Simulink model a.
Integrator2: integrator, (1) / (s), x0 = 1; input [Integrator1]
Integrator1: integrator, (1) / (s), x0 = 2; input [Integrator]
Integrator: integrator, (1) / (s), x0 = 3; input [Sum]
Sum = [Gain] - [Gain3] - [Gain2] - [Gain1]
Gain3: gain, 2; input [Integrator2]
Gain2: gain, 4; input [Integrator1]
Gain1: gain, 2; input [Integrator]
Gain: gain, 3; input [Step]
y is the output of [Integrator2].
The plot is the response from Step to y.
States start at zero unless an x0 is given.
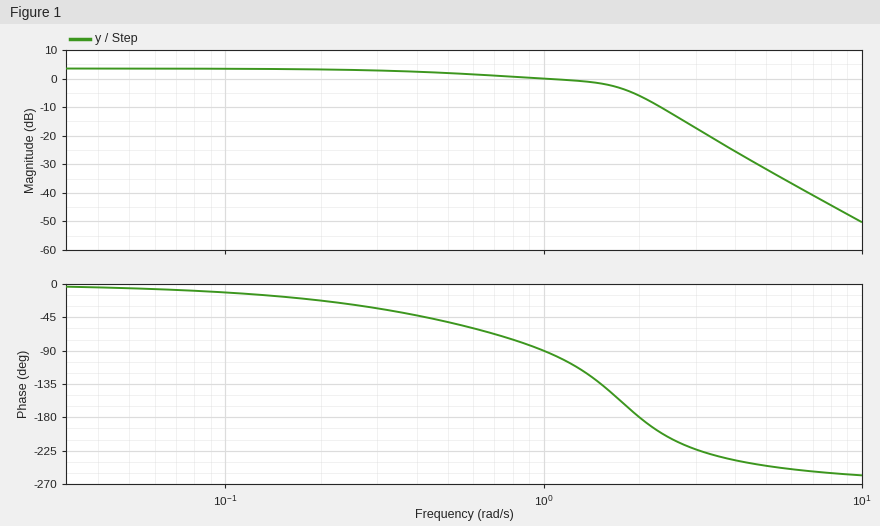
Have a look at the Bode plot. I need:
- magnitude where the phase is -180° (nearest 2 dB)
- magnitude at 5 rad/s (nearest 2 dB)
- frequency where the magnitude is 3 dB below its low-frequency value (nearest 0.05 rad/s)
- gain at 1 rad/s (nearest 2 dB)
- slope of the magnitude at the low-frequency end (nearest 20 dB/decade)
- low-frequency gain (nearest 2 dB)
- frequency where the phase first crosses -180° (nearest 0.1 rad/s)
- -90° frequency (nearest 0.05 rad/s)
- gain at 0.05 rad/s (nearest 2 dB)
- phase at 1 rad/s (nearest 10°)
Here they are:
-6 dB
-32 dB
0.85 rad/s
0 dB
0 dB/decade
4 dB
2.0 rad/s
1.00 rad/s
4 dB
-90°
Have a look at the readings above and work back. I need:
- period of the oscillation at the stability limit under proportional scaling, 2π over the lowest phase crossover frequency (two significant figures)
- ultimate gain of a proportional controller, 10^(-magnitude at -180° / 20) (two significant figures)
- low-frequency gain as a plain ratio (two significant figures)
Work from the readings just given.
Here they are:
3.1 s
2.0
1.6
